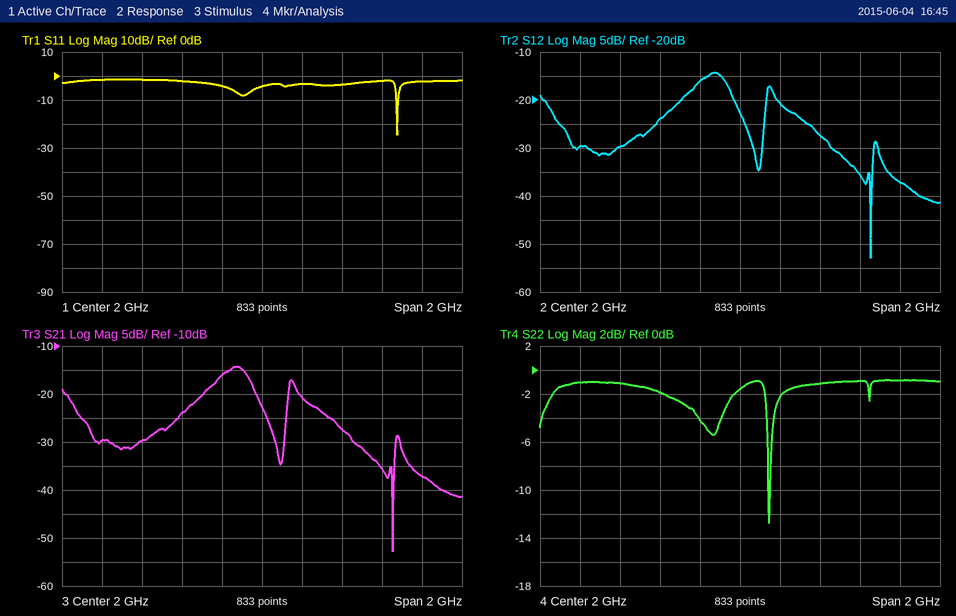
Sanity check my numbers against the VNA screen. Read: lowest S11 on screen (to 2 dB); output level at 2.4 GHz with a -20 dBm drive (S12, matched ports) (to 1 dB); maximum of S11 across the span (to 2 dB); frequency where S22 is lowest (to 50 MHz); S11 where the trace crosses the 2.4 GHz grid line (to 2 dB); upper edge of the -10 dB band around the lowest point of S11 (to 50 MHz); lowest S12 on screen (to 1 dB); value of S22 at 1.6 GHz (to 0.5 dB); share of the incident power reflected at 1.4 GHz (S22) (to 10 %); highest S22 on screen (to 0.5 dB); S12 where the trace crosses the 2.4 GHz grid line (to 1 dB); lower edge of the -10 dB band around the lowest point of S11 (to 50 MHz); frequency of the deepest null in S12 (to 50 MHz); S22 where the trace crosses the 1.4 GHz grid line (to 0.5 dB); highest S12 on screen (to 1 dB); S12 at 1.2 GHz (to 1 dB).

-24 dB
-47 dBm
-2 dB
2.15 GHz
-4 dB
2.70 GHz
-53 dB
-2.0 dB
80 %
-1.0 dB
-27 dB
2.65 GHz
2.65 GHz
-1.0 dB
-14 dB
-30 dB
